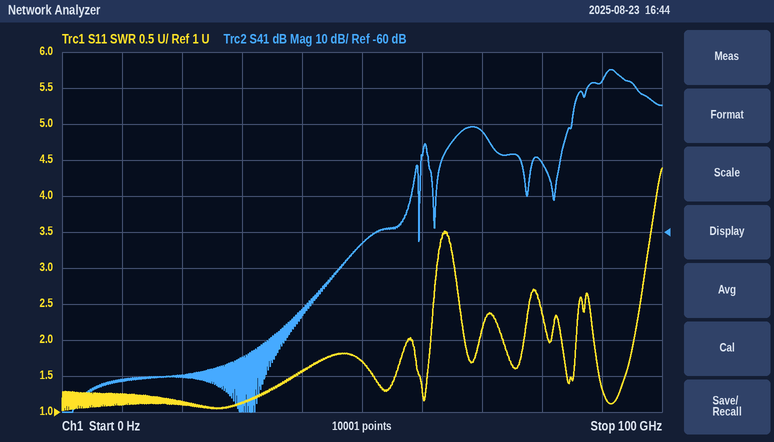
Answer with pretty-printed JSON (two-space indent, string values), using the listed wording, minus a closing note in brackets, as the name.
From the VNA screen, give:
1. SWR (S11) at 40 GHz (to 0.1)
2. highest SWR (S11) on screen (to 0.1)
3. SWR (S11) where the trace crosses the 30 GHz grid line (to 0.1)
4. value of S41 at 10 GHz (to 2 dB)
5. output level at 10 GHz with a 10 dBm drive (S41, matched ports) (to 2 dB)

{
  "SWR (S11) at 40 GHz": "1.6",
  "highest SWR (S11) on screen": "4.4",
  "SWR (S11) where the trace crosses the 30 GHz grid line": "1.1",
  "value of S41 at 10 GHz": "-102 dB",
  "output level at 10 GHz with a 10 dBm drive (S41, matched ports)": "-92 dBm"
}
